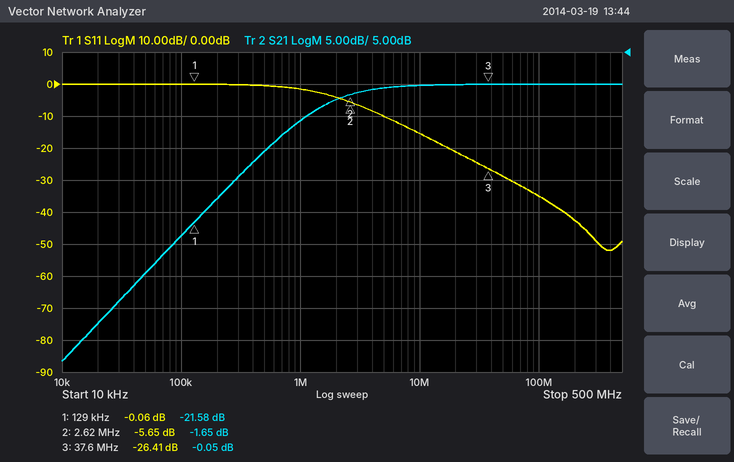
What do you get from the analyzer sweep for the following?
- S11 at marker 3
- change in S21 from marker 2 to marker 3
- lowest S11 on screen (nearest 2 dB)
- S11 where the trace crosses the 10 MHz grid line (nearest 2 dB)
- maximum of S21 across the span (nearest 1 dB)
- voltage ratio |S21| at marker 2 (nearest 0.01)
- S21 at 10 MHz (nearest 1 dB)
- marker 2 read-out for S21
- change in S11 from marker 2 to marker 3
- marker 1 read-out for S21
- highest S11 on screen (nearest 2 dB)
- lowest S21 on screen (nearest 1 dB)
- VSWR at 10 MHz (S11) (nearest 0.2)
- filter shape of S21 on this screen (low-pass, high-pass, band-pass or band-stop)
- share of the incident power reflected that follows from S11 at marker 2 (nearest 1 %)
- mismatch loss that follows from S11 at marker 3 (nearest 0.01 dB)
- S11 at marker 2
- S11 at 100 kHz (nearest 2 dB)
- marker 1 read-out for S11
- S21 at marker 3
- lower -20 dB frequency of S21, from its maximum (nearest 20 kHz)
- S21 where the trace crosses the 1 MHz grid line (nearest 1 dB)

-26.41 dB
1.60 dB
-52 dB
-16 dB
0 dB
0.83
0 dB
-1.65 dB
-20.76 dB
-21.58 dB
0 dB
-43 dB
1.4
high-pass
27 %
0.01 dB
-5.65 dB
0 dB
-0.06 dB
-0.05 dB
160 kHz
-6 dB
